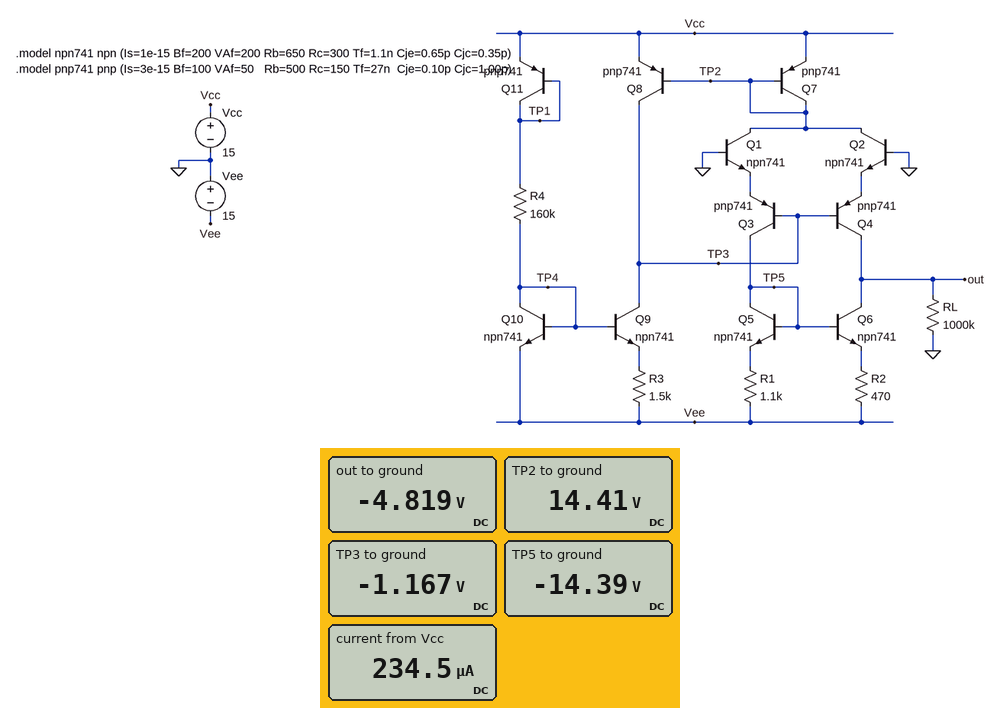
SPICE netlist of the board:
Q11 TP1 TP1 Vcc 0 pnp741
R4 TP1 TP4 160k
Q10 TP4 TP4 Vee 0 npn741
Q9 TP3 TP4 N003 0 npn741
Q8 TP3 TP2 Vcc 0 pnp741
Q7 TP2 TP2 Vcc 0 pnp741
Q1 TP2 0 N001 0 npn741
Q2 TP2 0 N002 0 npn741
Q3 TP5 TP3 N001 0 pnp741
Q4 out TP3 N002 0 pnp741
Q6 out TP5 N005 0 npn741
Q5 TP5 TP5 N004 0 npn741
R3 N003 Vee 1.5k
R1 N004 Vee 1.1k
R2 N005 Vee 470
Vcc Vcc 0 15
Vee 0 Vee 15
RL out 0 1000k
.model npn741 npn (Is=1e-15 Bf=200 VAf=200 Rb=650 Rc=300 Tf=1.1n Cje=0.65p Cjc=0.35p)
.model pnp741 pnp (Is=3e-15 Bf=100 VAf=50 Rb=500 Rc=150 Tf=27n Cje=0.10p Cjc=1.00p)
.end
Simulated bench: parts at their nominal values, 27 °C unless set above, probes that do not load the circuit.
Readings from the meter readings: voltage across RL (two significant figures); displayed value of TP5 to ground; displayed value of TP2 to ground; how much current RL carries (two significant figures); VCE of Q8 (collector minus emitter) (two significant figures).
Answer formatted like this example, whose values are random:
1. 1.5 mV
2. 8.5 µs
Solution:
1. 4.8 V
2. -14.39 V
3. 14.41 V
4. 4.8 µA
5. -16 V
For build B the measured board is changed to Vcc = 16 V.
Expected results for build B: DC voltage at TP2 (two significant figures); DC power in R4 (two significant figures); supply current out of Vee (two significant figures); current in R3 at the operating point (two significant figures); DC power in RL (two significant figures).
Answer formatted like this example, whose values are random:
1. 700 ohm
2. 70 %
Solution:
1. 15 V
2. 5.5 mW
3. 250 µA
4. 32 µA
5. 23 µW
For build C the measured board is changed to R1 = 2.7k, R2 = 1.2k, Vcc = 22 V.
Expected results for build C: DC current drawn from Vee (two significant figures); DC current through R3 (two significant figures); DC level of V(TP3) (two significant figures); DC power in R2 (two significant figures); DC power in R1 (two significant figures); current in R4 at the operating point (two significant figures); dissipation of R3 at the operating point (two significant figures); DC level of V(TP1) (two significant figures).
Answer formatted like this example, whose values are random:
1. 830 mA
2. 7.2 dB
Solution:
1. 290 µA
2. 34 µA
3. -1.2 V
4. 410 nW
5. 390 nW
6. 220 µA
7. 1.7 µW
8. 21 V
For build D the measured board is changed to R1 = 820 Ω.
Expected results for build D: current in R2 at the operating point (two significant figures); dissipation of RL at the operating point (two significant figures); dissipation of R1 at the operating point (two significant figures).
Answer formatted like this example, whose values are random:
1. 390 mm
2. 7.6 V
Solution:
1. 15 µA
2. 12 µW
3. 130 nW
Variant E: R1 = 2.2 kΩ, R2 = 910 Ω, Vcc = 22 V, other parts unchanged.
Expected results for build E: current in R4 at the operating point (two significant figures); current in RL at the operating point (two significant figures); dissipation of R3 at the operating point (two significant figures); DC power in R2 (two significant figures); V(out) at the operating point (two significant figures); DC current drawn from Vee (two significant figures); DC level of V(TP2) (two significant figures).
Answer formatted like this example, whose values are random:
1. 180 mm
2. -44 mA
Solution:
1. 220 µA
2. 6.8 µA
3. 1.7 µW
4. 300 nW
5. -6.8 V
6. 290 µA
7. 21 V
